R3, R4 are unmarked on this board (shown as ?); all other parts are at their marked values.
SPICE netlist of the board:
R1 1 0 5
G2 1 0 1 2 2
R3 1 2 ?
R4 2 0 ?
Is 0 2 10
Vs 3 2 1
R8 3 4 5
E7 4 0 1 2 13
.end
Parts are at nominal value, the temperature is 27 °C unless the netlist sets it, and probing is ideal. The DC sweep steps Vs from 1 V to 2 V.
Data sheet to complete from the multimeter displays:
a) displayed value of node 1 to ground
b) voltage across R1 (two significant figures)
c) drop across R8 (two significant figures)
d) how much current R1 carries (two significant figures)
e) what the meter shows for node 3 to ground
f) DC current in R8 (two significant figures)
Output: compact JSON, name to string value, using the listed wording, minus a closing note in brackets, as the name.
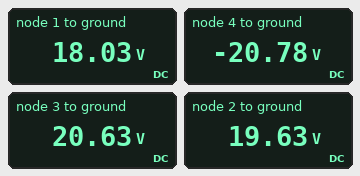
{"displayed value of node 1 to ground": "18.03 V", "voltage across R1": "18 V", "drop across R8": "41 V", "how much current R1 carries": "3.6 A", "what the meter shows for node 3 to ground": "20.63 V", "DC current in R8": "8.3 A"}
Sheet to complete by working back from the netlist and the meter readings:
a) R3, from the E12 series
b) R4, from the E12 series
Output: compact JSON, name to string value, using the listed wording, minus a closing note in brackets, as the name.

{"R3, from the E12 series": "3.9 Ω", "R4, from the E12 series": "15 Ω"}
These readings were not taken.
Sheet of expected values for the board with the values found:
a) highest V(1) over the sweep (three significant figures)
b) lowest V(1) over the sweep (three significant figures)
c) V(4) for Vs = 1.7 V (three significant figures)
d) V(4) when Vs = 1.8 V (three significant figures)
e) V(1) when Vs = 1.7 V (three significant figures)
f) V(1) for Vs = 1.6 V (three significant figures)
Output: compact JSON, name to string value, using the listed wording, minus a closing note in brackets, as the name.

{"highest V(1) over the sweep": "18.0 V", "lowest V(1) over the sweep": "17.7 V", "V(4) for Vs = 1.7 V": "-20.5 V", "V(4) when Vs = 1.8 V": "-20.4 V", "V(1) when Vs = 1.7 V": "17.8 V", "V(1) for Vs = 1.6 V": "17.8 V"}
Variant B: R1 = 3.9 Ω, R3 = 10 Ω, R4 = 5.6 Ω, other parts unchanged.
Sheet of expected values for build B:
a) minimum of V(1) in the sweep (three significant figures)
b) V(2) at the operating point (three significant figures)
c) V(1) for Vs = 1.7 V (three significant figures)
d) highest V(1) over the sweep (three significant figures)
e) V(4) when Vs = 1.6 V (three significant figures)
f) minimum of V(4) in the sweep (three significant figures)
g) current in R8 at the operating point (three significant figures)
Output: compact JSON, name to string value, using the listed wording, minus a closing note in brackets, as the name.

{"minimum of V(1) in the sweep": "12.7 V", "V(2) at the operating point": "14.6 V", "V(1) for Vs = 1.7 V": "12.8 V", "highest V(1) over the sweep": "13.0 V", "V(4) when Vs = 1.6 V": "-20.4 V", "minimum of V(4) in the sweep": "-20.6 V", "current in R8 at the operating point": "7.24 A"}
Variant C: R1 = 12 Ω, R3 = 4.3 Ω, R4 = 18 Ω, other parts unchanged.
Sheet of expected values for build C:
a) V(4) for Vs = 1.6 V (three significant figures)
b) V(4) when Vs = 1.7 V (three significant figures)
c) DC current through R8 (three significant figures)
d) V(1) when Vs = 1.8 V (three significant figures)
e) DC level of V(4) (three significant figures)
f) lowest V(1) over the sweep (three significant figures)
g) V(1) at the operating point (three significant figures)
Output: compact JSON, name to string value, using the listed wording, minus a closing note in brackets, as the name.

{"V(4) for Vs = 1.6 V": "-12.7 V", "V(4) when Vs = 1.7 V": "-12.6 V", "DC current through R8": "8.25 A", "V(1) when Vs = 1.8 V": "26.0 V", "DC level of V(4)": "-12.8 V", "lowest V(1) over the sweep": "25.9 V", "V(1) at the operating point": "26.4 V"}
